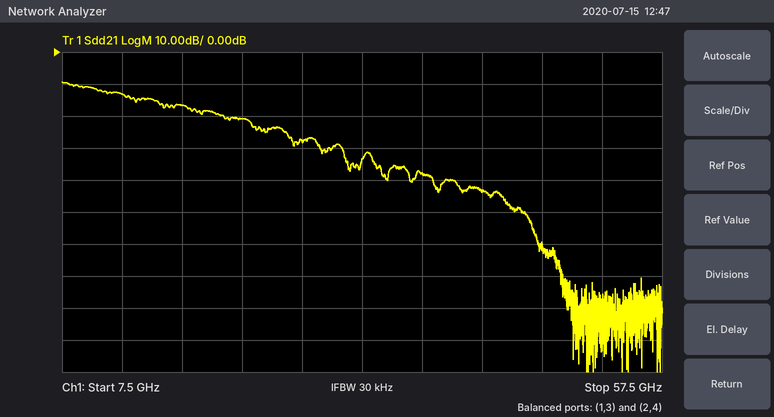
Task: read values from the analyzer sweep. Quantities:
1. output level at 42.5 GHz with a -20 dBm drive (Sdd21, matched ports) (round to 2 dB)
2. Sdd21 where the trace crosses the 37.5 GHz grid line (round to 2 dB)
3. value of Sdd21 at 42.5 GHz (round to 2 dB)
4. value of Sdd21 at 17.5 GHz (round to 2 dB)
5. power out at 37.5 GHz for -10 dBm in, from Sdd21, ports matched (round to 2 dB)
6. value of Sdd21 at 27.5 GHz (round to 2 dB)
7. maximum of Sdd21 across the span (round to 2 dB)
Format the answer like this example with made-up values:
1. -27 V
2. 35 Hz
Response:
1. -64 dBm
2. -38 dB
3. -44 dB
4. -16 dB
5. -48 dBm
6. -28 dB
7. -10 dB
